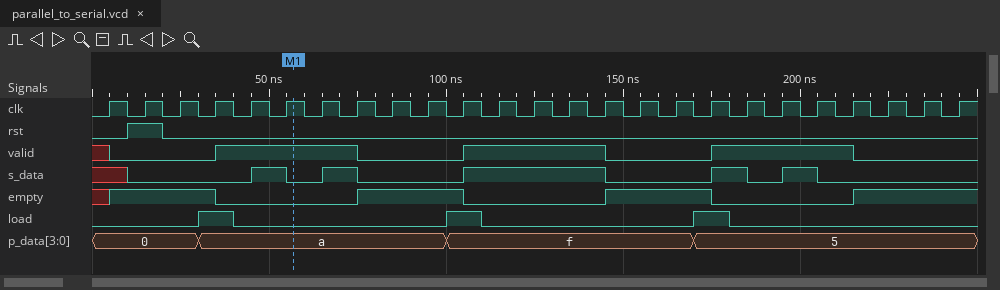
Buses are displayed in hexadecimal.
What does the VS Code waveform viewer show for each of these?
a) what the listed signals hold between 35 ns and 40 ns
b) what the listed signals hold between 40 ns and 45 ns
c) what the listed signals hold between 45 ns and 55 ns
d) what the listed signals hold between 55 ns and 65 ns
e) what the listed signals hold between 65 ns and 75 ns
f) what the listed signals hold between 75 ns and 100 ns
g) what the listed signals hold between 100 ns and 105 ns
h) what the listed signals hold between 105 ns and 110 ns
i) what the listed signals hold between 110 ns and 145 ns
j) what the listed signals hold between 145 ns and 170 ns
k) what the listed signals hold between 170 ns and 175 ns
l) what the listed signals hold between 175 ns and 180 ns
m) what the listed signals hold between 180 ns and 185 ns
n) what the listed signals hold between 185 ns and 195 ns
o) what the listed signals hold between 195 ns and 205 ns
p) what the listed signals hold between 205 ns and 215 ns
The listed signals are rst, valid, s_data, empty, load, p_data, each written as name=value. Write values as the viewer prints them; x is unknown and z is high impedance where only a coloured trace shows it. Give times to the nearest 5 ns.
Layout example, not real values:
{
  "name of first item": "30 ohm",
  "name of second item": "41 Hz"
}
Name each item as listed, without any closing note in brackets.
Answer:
{
  "what the listed signals hold between 35 ns and 40 ns": "rst=0, valid=1, s_data=0, empty=0, load=1, p_data=a",
  "what the listed signals hold between 40 ns and 45 ns": "rst=0, valid=1, s_data=0, empty=0, load=0, p_data=a",
  "what the listed signals hold between 45 ns and 55 ns": "rst=0, valid=1, s_data=1, empty=0, load=0, p_data=a",
  "what the listed signals hold between 55 ns and 65 ns": "rst=0, valid=1, s_data=0, empty=0, load=0, p_data=a",
  "what the listed signals hold between 65 ns and 75 ns": "rst=0, valid=1, s_data=1, empty=0, load=0, p_data=a",
  "what the listed signals hold between 75 ns and 100 ns": "rst=0, valid=0, s_data=0, empty=1, load=0, p_data=a",
  "what the listed signals hold between 100 ns and 105 ns": "rst=0, valid=0, s_data=0, empty=1, load=1, p_data=f",
  "what the listed signals hold between 105 ns and 110 ns": "rst=0, valid=1, s_data=1, empty=0, load=1, p_data=f",
  "what the listed signals hold between 110 ns and 145 ns": "rst=0, valid=1, s_data=1, empty=0, load=0, p_data=f",
  "what the listed signals hold between 145 ns and 170 ns": "rst=0, valid=0, s_data=0, empty=1, load=0, p_data=f",
  "what the listed signals hold between 170 ns and 175 ns": "rst=0, valid=0, s_data=0, empty=1, load=1, p_data=5",
  "what the listed signals hold between 175 ns and 180 ns": "rst=0, valid=1, s_data=1, empty=0, load=1, p_data=5",
  "what the listed signals hold between 180 ns and 185 ns": "rst=0, valid=1, s_data=1, empty=0, load=0, p_data=5",
  "what the listed signals hold between 185 ns and 195 ns": "rst=0, valid=1, s_data=0, empty=0, load=0, p_data=5",
  "what the listed signals hold between 195 ns and 205 ns": "rst=0, valid=1, s_data=1, empty=0, load=0, p_data=5",
  "what the listed signals hold between 205 ns and 215 ns": "rst=0, valid=1, s_data=0, empty=0, load=0, p_data=5"
}
